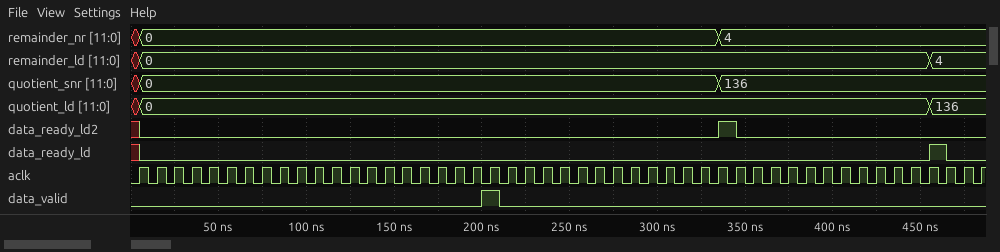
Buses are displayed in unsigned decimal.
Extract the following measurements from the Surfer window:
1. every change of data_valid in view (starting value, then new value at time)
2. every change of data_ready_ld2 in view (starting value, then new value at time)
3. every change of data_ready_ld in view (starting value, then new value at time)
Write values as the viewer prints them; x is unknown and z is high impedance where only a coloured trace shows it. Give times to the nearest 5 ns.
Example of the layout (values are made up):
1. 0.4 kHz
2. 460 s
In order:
1. 0, 1 at 200 ns, 0 at 210 ns
2. x, 0 at 5 ns, 1 at 335 ns, 0 at 345 ns
3. x, 0 at 5 ns, 1 at 455 ns, 0 at 465 ns
